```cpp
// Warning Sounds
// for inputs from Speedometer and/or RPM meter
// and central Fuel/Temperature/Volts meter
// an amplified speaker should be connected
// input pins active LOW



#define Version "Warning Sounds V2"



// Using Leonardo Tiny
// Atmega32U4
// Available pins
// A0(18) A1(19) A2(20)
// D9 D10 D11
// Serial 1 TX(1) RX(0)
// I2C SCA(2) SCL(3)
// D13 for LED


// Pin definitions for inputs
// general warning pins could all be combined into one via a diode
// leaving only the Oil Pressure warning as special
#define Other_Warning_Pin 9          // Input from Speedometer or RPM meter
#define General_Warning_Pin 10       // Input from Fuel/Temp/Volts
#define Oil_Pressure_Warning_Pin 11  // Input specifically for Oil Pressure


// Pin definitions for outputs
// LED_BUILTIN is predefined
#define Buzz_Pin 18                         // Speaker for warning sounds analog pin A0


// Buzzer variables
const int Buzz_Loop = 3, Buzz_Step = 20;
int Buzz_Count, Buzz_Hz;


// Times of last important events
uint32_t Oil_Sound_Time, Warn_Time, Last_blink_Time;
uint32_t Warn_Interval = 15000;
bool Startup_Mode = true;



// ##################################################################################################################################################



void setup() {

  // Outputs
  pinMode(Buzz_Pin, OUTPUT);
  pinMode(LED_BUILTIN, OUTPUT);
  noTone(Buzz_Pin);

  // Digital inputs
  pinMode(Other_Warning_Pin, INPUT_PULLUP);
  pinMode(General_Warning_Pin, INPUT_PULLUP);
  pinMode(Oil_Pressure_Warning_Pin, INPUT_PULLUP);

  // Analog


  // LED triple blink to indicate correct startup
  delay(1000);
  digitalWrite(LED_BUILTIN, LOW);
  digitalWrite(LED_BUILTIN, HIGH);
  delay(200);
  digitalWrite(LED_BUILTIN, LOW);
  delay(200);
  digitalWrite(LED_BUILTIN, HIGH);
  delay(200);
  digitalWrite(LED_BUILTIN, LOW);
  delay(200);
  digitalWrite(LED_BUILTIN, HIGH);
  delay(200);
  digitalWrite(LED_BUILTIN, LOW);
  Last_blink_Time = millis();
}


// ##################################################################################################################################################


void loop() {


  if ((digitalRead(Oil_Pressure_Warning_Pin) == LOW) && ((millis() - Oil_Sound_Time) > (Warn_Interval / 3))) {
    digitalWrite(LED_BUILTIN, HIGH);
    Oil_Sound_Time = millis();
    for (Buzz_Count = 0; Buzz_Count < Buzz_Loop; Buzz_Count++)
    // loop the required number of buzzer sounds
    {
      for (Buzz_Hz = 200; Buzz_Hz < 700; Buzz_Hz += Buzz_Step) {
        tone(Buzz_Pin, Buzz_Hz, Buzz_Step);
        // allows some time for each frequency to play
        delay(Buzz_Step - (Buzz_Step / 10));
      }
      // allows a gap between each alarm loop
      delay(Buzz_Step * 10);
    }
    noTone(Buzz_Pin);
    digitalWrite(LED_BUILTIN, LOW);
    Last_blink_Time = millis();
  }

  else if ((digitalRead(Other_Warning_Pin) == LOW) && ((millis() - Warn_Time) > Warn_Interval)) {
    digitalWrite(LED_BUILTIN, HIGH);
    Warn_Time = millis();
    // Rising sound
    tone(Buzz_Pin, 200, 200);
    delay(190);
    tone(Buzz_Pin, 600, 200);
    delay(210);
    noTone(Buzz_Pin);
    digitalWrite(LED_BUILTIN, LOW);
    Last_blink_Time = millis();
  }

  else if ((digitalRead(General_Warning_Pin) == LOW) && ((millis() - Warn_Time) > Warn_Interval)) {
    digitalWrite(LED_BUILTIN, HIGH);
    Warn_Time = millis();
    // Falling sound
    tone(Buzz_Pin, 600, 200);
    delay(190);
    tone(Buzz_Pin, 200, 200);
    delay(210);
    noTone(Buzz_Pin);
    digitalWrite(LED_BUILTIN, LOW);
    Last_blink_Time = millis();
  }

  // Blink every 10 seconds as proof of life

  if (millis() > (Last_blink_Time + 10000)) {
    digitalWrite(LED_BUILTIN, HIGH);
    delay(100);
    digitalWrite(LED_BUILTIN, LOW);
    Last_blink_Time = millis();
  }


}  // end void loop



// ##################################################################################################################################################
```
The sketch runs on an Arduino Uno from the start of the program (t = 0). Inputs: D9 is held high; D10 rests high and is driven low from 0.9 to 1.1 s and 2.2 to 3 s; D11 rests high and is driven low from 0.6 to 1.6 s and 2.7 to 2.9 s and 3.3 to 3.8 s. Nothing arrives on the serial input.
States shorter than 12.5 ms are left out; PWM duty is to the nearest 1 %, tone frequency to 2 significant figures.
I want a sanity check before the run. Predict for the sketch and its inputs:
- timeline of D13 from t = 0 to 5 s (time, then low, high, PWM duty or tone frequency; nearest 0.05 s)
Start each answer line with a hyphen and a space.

- 0 s low; 1 s high; 1.2 s low; 1.4 s high; 1.6 s low; 1.8 s high; 2 s low
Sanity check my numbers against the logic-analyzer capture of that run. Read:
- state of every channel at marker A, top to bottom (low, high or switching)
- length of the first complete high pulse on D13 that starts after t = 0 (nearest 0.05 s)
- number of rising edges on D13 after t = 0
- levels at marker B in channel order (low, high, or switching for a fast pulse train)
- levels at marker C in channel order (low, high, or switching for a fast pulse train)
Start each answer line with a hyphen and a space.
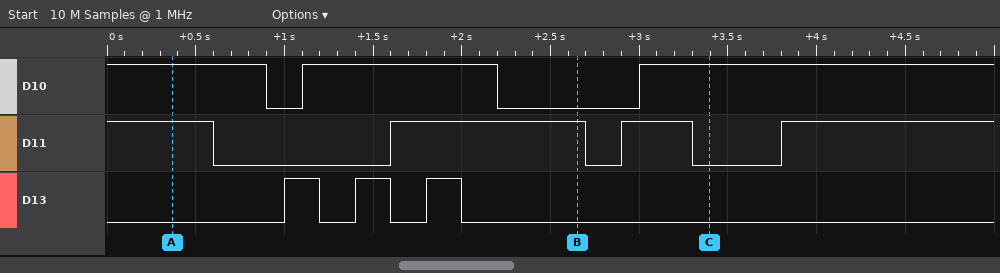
- D10 high, D11 high, D13 low
- 0.20 s
- 3
- D10 low, D11 high, D13 low
- D10 high, D11 low, D13 low
